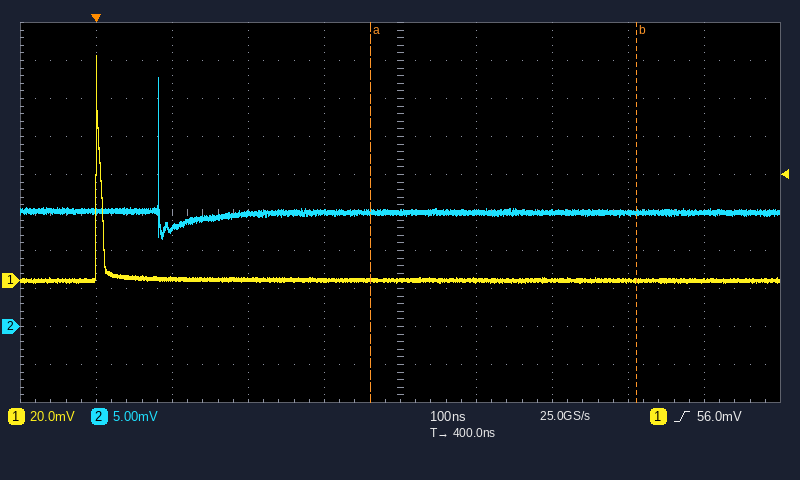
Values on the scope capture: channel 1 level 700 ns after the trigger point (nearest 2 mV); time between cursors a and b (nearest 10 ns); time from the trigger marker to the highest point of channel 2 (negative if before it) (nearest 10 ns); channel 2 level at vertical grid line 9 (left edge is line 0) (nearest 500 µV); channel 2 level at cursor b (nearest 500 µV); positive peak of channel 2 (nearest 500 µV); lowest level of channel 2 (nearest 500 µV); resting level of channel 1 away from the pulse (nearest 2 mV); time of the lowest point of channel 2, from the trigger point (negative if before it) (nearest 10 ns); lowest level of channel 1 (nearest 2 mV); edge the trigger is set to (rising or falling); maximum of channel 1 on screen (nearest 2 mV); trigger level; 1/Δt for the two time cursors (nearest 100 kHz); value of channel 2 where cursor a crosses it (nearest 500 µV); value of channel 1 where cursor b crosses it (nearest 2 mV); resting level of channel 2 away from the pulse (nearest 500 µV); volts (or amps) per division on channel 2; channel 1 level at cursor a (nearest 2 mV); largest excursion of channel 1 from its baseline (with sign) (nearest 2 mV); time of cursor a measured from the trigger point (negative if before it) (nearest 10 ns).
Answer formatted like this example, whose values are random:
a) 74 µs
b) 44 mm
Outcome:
a) 0 mV
b) 350 ns
c) +80 ns
d) 15.0 mV
e) 15.0 mV
f) 33.0 mV
g) 11.5 mV
h) 0 mV
i) +90 ns
j) 0 mV
k) rising
l) 118 mV
m) 56.0 mV
n) 2.9 MHz
o) 15.0 mV
p) 0 mV
q) 15.0 mV
r) 5 mV
s) 0 mV
t) +118 mV
u) +360 ns
